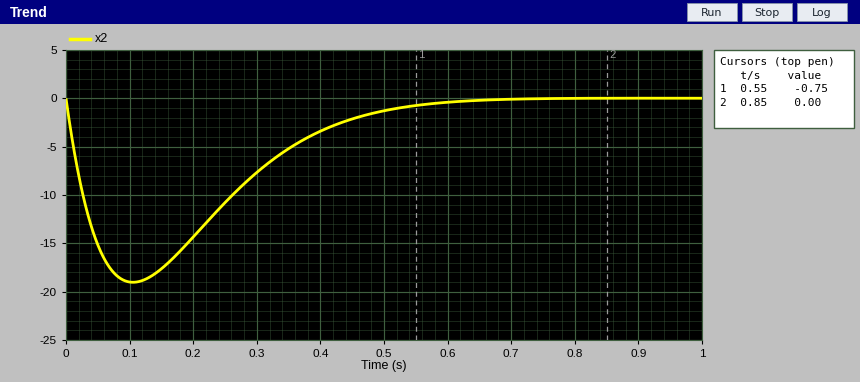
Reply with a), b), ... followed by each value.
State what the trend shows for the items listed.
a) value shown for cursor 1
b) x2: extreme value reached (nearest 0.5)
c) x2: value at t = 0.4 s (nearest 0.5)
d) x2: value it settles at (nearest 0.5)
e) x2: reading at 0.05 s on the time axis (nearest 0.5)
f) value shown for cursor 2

a) -0.75
b) -19.0
c) -3.5
d) 0.0
e) -15.0
f) 0.00
